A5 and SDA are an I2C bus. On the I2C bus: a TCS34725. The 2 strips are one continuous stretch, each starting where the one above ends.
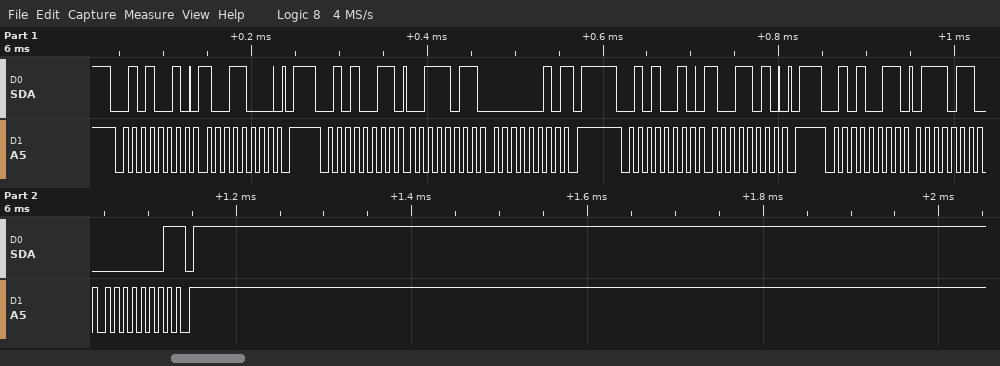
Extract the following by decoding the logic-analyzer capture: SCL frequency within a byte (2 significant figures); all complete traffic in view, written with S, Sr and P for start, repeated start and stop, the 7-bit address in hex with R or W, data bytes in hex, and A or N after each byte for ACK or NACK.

100 kHz
S 29W A 98 A P S 29R A 3B A 02 N P S 29W A 9A A P S 29R A 76 A 01 N P
